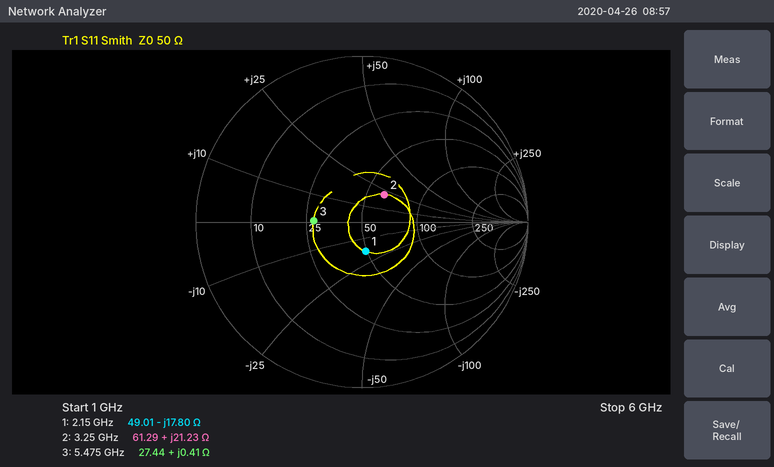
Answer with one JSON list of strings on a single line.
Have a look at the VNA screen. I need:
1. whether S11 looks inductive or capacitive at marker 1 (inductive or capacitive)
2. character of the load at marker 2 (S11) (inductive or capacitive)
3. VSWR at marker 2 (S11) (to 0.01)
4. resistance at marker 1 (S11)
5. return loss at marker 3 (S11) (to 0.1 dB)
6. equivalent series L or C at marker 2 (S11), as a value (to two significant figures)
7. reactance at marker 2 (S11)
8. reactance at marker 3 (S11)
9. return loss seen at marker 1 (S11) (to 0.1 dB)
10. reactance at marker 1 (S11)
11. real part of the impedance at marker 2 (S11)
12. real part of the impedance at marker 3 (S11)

["capacitive", "inductive", "1.54", "49.01 Ω", "10.7 dB", "1.0 nH", "+21.23 Ω", "+0.41 Ω", "15.0 dB", "-17.80 Ω", "61.29 Ω", "27.44 Ω"]
